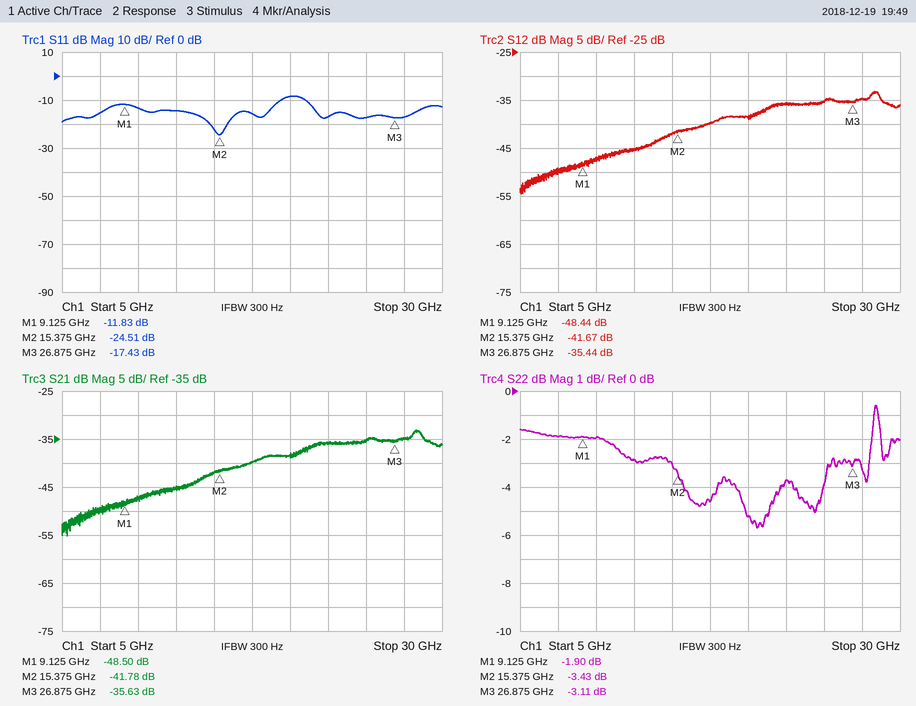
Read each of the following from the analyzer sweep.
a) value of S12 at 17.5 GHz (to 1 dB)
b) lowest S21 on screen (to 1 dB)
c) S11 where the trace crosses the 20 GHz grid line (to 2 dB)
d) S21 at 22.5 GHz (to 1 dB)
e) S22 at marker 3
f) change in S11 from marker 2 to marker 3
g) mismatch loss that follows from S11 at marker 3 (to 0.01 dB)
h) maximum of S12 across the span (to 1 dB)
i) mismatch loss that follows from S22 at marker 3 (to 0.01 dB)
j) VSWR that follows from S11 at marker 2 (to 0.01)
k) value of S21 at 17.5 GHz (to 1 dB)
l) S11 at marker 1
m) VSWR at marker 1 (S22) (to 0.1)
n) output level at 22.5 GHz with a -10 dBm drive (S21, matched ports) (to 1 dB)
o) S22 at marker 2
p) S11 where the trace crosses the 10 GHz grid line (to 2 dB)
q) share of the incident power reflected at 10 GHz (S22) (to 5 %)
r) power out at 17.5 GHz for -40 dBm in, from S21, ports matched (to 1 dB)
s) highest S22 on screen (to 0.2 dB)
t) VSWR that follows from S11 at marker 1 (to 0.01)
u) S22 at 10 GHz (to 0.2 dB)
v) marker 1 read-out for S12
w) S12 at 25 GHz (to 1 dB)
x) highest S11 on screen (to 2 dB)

-40 dB
-55 dB
-8 dB
-36 dB
-3.11 dB
7.08 dB
0.08 dB
-33 dB
2.91 dB
1.13
-40 dB
-11.83 dB
9.2
-46 dBm
-3.43 dB
-14 dB
65 %
-80 dBm
-0.6 dB
1.69
-2.0 dB
-48.44 dB
-35 dB
-8 dB
